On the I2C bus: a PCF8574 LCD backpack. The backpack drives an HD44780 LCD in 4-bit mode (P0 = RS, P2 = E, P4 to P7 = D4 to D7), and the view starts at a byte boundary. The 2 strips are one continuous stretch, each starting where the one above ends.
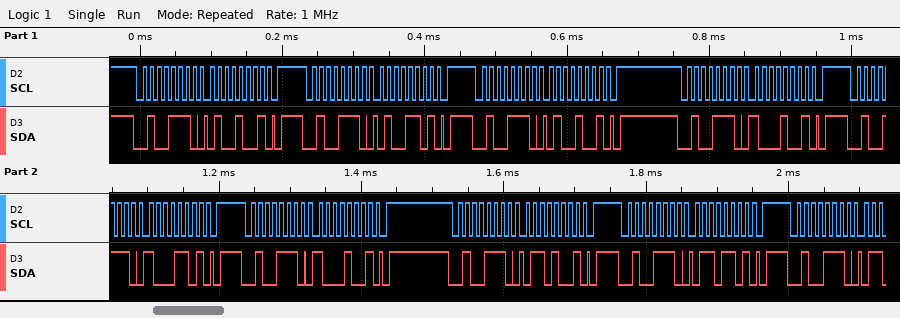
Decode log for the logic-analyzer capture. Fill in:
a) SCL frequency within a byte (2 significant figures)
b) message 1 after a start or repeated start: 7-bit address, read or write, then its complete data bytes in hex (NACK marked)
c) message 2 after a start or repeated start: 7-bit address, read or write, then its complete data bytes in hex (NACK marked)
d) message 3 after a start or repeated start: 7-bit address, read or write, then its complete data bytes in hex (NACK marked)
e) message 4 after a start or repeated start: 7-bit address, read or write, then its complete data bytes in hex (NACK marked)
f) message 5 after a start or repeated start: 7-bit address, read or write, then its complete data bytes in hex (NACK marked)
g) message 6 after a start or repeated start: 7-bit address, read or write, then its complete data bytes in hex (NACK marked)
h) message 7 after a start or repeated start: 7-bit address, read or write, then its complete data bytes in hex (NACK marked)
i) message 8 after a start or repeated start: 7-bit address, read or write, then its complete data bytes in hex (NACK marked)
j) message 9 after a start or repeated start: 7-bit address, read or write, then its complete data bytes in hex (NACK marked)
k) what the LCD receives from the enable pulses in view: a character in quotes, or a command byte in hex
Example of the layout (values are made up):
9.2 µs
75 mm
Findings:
100 kHz
0x27 write: 49
0x27 write: 4D
0x27 write: 49
0x27 write: 89
0x27 write: 8D
0x27 write: 89
0x27 write: 69
0x27 write: 6D
0x27 write
'H'
